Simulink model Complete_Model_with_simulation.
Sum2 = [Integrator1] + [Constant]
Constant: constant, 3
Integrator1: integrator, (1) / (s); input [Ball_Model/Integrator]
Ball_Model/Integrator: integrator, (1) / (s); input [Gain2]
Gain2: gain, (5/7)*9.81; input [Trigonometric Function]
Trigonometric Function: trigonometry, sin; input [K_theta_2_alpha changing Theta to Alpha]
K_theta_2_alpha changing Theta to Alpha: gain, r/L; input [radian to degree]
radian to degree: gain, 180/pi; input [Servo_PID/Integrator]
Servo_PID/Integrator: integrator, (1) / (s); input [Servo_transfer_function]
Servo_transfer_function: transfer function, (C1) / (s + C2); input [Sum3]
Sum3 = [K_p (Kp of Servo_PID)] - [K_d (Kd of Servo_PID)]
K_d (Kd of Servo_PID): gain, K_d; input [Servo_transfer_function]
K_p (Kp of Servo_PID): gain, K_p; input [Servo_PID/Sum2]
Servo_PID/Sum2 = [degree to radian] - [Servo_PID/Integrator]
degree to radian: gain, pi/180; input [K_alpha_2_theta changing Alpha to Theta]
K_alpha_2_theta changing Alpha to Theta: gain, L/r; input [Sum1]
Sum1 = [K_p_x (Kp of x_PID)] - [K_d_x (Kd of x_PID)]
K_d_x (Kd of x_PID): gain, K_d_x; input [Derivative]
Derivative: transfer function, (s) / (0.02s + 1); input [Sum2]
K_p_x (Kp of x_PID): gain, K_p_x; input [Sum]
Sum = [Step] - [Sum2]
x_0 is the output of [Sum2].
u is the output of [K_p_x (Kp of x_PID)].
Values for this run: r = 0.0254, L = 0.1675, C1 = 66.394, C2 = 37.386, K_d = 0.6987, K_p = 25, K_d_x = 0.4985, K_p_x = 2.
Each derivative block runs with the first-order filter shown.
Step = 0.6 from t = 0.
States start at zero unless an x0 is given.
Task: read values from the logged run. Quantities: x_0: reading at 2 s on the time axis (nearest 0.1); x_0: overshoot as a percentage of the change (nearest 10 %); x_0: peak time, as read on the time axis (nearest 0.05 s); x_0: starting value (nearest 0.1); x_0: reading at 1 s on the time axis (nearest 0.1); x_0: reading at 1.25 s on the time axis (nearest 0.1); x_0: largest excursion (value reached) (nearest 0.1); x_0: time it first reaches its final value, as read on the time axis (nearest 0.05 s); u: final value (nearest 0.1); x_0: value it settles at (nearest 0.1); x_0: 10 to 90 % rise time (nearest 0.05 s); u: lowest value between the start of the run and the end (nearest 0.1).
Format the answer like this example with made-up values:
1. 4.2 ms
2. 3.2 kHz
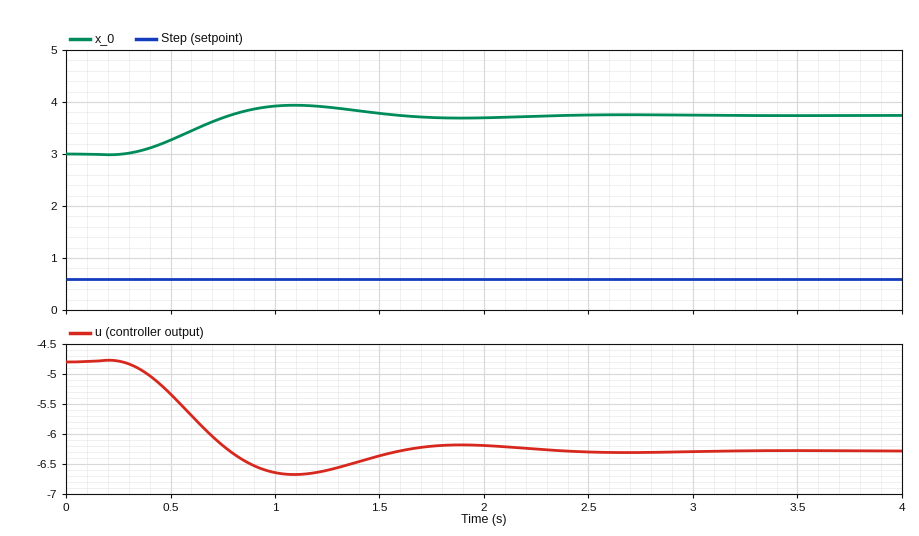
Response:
1. 3.7
2. 30 %
3. 1.10 s
4. 3.0
5. 3.9
6. 3.9
7. 3.9
8. 0.80 s
9. -6.3
10. 3.7
11. 0.35 s
12. -6.7
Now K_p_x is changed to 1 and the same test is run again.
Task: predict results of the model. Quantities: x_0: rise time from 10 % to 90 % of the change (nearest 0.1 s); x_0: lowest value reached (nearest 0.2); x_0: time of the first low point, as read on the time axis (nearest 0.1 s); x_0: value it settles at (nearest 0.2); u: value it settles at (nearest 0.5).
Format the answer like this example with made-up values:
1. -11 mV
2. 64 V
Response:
1. 0.7 s
2. 0.4
3. 1.9 s
4. 0.6
5. 0.0
